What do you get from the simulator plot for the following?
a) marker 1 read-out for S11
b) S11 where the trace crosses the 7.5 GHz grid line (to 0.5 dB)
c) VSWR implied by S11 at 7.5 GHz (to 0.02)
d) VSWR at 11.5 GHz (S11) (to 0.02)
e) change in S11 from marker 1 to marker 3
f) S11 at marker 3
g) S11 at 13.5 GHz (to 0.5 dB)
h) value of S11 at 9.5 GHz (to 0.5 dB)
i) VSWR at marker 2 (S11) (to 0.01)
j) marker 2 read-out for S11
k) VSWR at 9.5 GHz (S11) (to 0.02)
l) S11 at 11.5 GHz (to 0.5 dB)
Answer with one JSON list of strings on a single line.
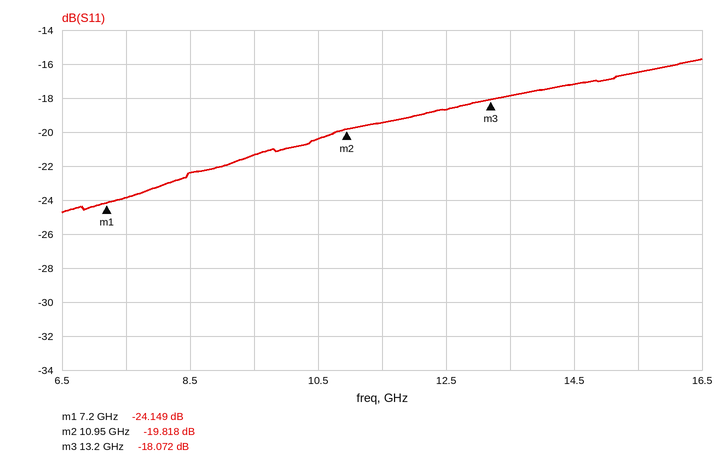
["-24.149 dB", "-24.0 dB", "1.14", "1.24", "6.077 dB", "-18.072 dB", "-18.0 dB", "-21.5 dB", "1.23", "-19.818 dB", "1.18", "-19.5 dB"]
